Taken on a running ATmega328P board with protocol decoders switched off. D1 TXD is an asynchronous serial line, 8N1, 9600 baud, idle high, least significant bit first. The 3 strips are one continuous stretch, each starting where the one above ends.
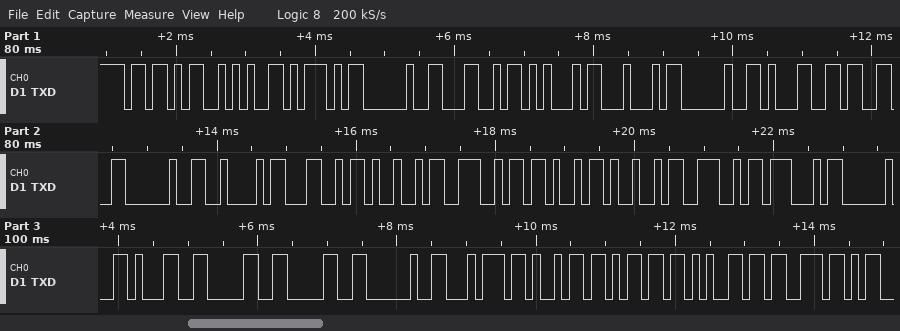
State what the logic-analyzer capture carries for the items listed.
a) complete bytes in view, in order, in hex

5B 2A 5D 20 4C 45 44 20 31 33 20 42 4C 49 4E 4B 49 4E 47 20 31 30 30 20 74 69 6D 65 73
